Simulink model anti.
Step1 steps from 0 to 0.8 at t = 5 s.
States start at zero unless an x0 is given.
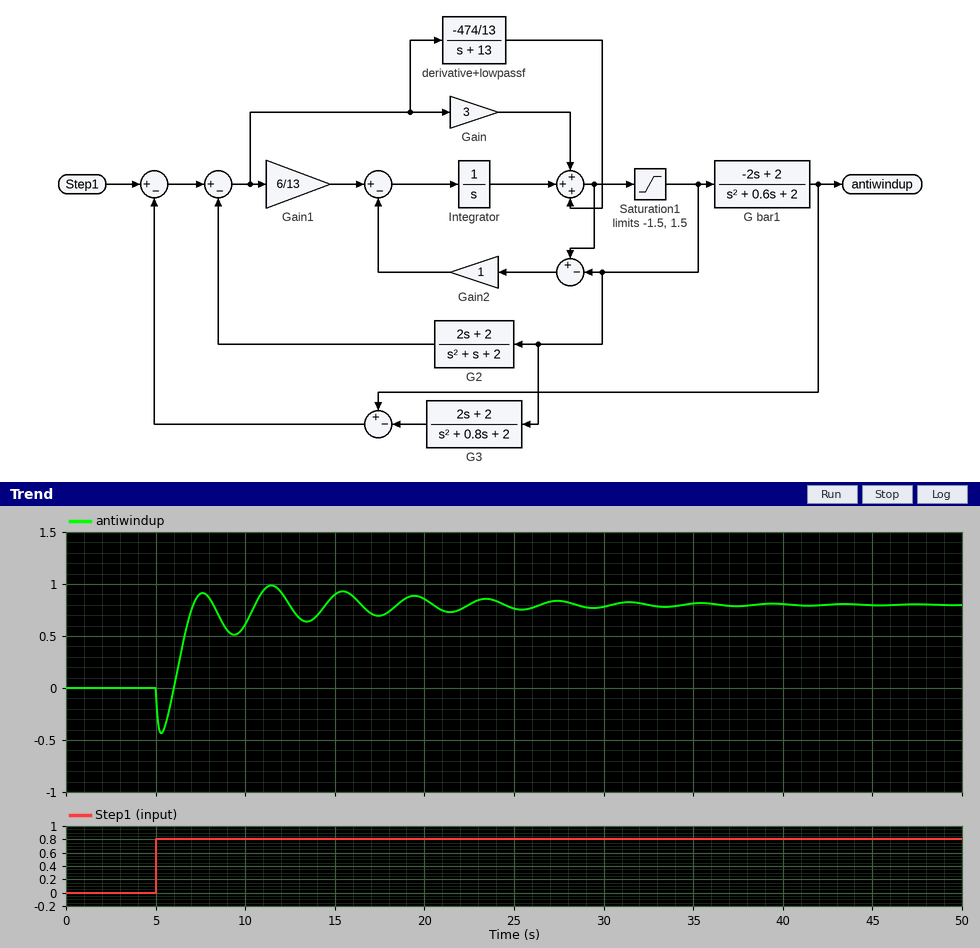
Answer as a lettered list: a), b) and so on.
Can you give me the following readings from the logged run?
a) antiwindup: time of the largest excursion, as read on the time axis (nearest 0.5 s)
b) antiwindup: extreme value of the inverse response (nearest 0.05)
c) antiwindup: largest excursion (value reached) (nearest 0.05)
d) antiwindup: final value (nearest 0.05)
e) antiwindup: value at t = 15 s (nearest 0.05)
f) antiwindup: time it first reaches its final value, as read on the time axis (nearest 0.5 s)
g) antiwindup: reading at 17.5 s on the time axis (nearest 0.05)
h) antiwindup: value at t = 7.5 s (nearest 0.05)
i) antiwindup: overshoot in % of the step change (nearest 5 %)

a) 11.5 s
b) -0.45
c) 1.00
d) 0.80
e) 0.90
f) 7.0 s
g) 0.70
h) 0.90
i) 25 %
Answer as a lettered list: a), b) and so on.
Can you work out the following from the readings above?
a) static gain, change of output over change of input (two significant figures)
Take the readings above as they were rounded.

a) 1.0
